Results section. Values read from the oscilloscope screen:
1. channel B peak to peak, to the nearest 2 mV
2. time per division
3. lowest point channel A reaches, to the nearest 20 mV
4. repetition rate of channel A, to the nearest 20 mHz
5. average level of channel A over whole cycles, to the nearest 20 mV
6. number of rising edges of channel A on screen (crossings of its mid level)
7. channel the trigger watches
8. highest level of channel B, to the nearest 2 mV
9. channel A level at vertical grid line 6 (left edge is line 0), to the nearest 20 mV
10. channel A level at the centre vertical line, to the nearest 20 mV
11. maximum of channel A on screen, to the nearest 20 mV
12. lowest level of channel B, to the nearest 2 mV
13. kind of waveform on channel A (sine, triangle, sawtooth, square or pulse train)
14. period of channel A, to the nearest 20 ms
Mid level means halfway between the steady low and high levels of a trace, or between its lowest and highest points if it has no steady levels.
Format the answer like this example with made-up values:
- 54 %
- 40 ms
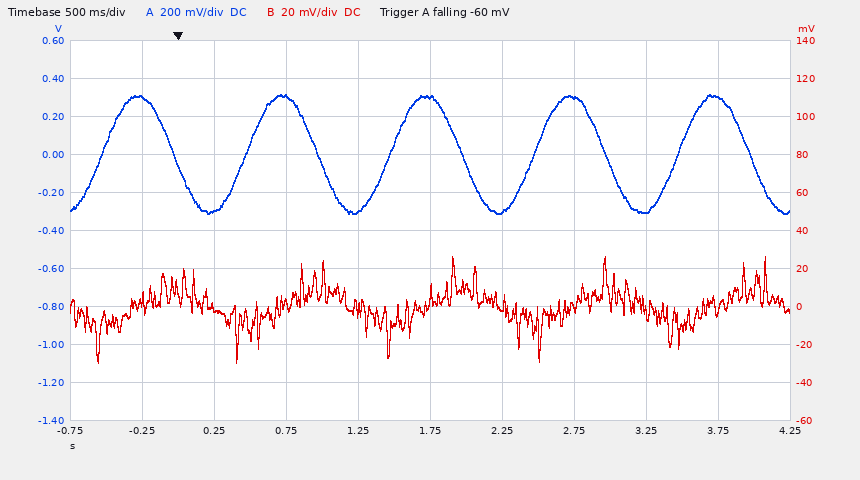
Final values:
- 56 mV
- 500 ms
- -320 mV
- 1.00 Hz
- 0 mV
- 5
- channel A
- 26 mV
- -300 mV
- 300 mV
- 320 mV
- -30 mV
- sine
- 1.00 s
